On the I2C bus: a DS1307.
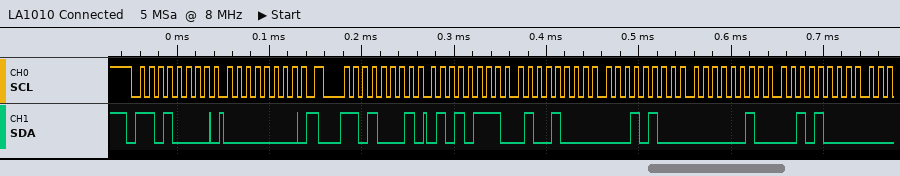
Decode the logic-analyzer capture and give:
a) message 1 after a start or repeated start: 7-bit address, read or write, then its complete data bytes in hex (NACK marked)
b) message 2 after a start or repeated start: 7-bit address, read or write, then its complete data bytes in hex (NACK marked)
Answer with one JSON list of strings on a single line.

["0x68 write: 00", "0x68 read: 57 48 14 02 28"]
